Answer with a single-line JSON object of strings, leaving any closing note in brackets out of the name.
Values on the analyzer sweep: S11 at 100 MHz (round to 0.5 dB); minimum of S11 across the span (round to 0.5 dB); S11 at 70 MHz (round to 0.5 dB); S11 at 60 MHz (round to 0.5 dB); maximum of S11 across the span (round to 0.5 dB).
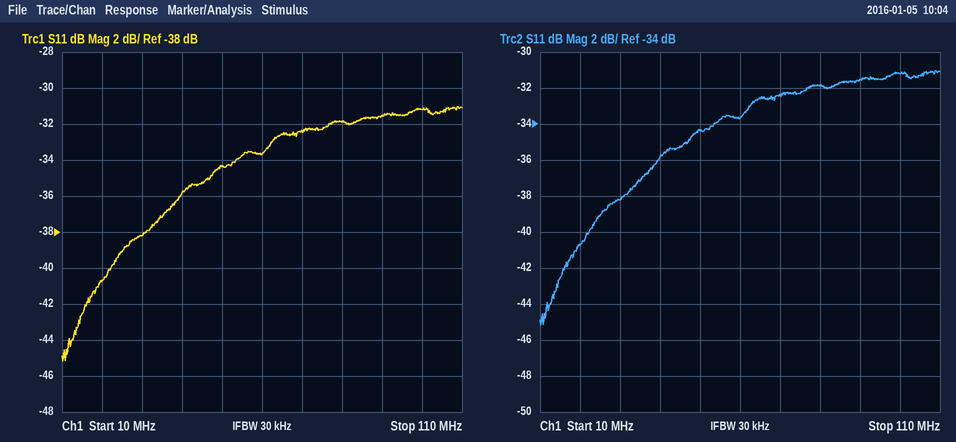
{"S11 at 100 MHz": "-31.0 dB", "minimum of S11 across the span": "-45.0 dB", "S11 at 70 MHz": "-32.5 dB", "S11 at 60 MHz": "-33.5 dB", "maximum of S11 across the span": "-31.0 dB"}
